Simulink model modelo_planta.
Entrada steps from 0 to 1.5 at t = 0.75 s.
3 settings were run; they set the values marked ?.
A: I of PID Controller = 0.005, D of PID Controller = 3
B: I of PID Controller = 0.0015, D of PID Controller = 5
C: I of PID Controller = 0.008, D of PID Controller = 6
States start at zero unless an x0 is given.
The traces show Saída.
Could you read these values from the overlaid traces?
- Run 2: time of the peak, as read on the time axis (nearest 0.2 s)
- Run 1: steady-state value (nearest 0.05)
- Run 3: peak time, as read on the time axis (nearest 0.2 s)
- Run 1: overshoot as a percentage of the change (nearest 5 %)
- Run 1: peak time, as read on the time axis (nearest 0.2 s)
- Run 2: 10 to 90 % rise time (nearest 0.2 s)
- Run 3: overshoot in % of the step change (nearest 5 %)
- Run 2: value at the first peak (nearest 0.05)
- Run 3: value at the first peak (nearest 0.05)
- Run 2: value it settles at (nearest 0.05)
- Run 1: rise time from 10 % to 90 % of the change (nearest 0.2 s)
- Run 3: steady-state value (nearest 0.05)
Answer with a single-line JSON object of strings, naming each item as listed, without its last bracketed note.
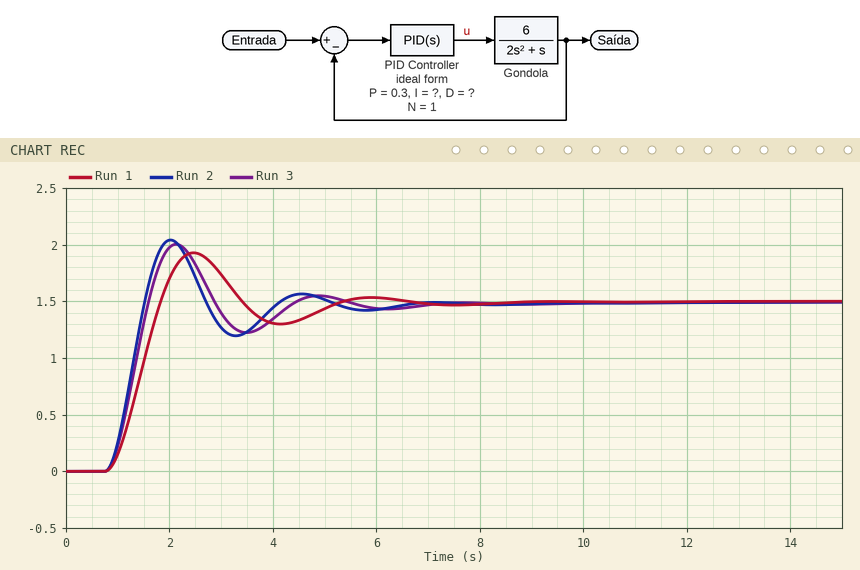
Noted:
{"Run 2: time of the peak, as read on the time axis": "2.0 s", "Run 1: steady-state value": "1.50", "Run 3: peak time, as read on the time axis": "2.2 s", "Run 1: overshoot as a percentage of the change": "30 %", "Run 1: peak time, as read on the time axis": "2.4 s", "Run 2: 10 to 90 % rise time": "0.6 s", "Run 3: overshoot in % of the step change": "35 %", "Run 2: value at the first peak": "2.05", "Run 3: value at the first peak": "2.00", "Run 2: value it settles at": "1.50", "Run 1: rise time from 10 % to 90 % of the change": "0.8 s", "Run 3: steady-state value": "1.50"}
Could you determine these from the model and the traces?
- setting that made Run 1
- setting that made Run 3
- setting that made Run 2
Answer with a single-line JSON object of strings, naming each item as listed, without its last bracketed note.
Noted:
{"setting that made Run 1": "A", "setting that made Run 3": "B", "setting that made Run 2": "C"}
